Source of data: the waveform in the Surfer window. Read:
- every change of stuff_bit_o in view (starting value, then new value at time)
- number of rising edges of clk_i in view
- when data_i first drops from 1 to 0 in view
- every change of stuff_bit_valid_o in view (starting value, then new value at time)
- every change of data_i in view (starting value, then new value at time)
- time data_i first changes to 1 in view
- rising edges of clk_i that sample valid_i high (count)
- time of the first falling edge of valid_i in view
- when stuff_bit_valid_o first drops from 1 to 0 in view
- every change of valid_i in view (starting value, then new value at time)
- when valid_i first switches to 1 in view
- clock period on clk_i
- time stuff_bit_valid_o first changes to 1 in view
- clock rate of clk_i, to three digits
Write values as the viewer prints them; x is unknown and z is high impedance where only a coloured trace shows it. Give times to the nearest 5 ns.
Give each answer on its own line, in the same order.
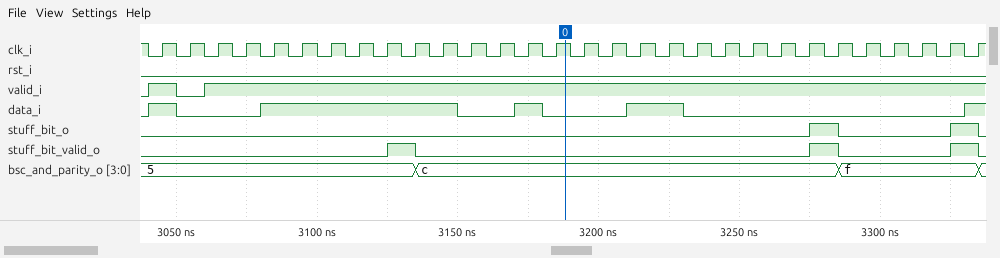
0, 1 at 3275 ns, 0 at 3285 ns, 1 at 3325 ns, 0 at 3335 ns
30
3050 ns
0, 1 at 3125 ns, 0 at 3135 ns, 1 at 3275 ns, 0 at 3285 ns, 1 at 3325 ns, 0 at 3335 ns
0, 1 at 3040 ns, 0 at 3050 ns, 1 at 3080 ns, 0 at 3150 ns, 1 at 3170 ns, 0 at 3180 ns, 1 at 3210 ns, 0 at 3230 ns, 1 at 3330 ns
3040 ns
29
3050 ns
3135 ns
0, 1 at 3040 ns, 0 at 3050 ns, 1 at 3060 ns
3040 ns
10 ns
3125 ns
100 MHz
